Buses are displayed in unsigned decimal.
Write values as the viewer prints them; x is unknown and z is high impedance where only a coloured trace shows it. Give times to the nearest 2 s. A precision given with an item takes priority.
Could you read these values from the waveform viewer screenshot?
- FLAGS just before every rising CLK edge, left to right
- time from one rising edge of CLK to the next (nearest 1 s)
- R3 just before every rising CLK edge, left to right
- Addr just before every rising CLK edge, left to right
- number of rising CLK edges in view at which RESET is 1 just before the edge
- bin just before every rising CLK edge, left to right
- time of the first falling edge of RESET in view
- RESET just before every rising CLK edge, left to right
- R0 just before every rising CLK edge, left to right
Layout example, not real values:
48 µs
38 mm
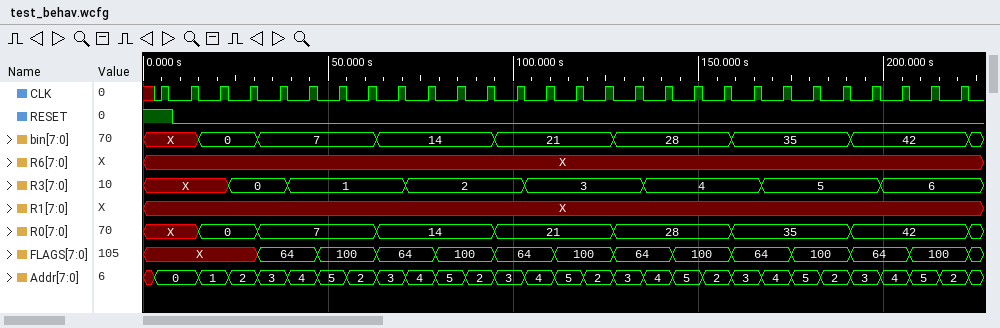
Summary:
X, X, X, X, 64, 64, 100, 100, 64, 64, 100, 100, 64, 64, 100, 100, 64, 64, 100, 100, 64, 64, 100, 100, 64, 64, 100, 100
8 s
X, X, X, 0, 0, 1, 1, 1, 1, 2, 2, 2, 2, 3, 3, 3, 3, 4, 4, 4, 4, 5, 5, 5, 5, 6, 6, 6
0, 0, 1, 2, 3, 4, 5, 2, 3, 4, 5, 2, 3, 4, 5, 2, 3, 4, 5, 2, 3, 4, 5, 2, 3, 4, 5, 2
1
X, X, 0, 0, 7, 7, 7, 7, 14, 14, 14, 14, 21, 21, 21, 21, 28, 28, 28, 28, 35, 35, 35, 35, 42, 42, 42, 42
8 s
1 0 0 0 0 0 0 0 0 0 0 0 0 0 0 0 0 0 0 0 0 0 0 0 0 0 0 0
X, X, 0, 0, 7, 7, 7, 7, 14, 14, 14, 14, 21, 21, 21, 21, 28, 28, 28, 28, 35, 35, 35, 35, 42, 42, 42, 42
